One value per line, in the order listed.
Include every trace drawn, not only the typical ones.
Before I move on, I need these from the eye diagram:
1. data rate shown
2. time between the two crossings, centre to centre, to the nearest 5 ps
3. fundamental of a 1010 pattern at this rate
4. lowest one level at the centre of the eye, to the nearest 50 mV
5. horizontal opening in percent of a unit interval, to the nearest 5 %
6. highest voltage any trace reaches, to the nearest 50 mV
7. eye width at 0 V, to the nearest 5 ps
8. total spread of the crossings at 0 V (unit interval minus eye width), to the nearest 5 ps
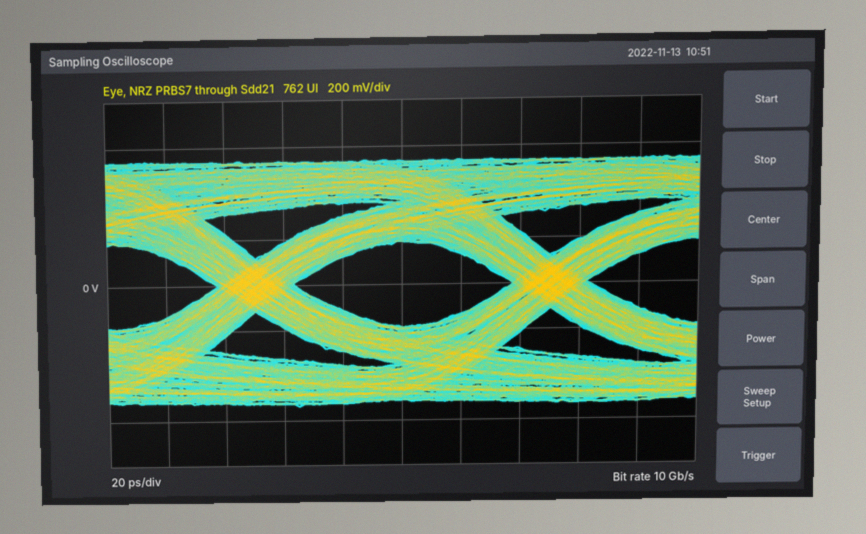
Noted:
10 Gb/s
100 ps
5 GHz
200 mV
75 %
550 mV
75 ps
25 ps
